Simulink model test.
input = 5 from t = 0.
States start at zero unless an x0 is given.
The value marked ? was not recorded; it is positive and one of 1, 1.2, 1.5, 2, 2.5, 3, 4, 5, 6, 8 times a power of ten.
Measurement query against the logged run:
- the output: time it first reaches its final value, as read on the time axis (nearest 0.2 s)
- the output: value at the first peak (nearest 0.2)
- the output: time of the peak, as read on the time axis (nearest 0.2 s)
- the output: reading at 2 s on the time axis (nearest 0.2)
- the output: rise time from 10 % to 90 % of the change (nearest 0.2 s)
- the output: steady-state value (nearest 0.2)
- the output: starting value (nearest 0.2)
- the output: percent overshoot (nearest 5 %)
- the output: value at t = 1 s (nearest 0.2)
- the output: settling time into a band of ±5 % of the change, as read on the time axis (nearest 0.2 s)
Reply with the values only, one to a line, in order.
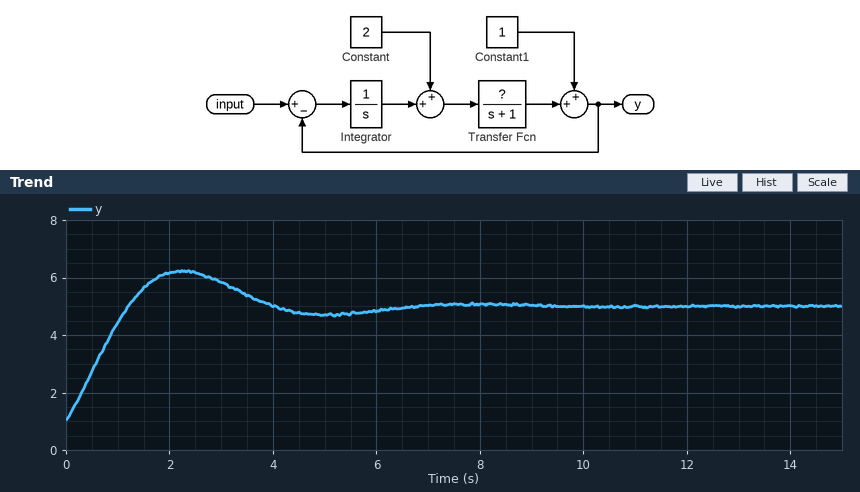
1.2 s
6.2
2.2 s
6.2
1.0 s
5.0
1.0
30 %
4.4
5.8 s
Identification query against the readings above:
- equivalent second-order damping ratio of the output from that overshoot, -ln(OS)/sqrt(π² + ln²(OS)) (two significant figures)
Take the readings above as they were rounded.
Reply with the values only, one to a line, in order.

0.36
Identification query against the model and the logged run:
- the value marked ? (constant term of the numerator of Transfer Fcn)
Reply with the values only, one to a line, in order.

1.5
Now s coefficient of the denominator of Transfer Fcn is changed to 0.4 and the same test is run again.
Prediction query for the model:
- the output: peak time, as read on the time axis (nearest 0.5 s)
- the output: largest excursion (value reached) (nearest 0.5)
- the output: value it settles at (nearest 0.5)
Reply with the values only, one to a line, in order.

1.5 s
5.5
5.0
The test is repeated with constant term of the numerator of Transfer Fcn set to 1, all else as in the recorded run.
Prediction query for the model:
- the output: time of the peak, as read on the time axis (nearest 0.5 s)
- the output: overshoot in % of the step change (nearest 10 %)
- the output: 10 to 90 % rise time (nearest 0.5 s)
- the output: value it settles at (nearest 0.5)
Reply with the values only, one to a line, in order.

3.0 s
20 %
1.5 s
5.0
